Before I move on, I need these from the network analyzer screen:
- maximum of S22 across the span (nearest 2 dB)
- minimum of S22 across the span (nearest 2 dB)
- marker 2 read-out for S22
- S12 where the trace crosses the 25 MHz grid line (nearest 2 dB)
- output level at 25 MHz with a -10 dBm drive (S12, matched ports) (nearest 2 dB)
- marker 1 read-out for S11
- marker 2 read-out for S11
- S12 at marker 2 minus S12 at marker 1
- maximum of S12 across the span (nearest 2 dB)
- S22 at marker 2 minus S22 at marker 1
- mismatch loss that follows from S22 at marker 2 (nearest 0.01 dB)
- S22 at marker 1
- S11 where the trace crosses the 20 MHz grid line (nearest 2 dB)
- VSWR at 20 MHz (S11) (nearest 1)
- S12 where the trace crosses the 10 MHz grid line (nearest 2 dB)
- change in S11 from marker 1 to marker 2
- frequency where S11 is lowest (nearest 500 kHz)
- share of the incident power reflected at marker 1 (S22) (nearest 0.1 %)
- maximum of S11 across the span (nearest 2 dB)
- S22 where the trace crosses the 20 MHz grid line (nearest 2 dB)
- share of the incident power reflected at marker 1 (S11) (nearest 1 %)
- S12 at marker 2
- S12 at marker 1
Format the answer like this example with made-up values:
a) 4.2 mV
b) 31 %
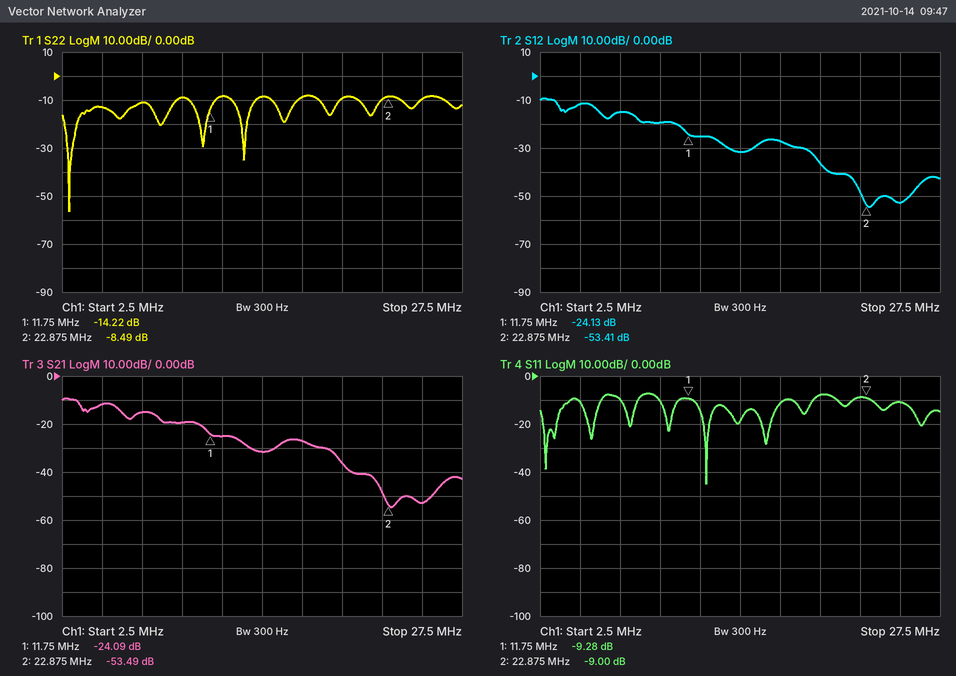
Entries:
a) -8 dB
b) -56 dB
c) -8.49 dB
d) -52 dB
e) -62 dBm
f) -9.28 dB
g) -9.00 dB
h) -29.28 dB
i) -10 dB
j) 5.73 dB
k) 0.66 dB
l) -14.22 dB
m) -8 dB
n) 2
o) -20 dB
p) 0.28 dB
q) 13.0 MHz
r) 3.8 %
s) -8 dB
t) -10 dB
u) 12 %
v) -53.41 dB
w) -24.13 dB
